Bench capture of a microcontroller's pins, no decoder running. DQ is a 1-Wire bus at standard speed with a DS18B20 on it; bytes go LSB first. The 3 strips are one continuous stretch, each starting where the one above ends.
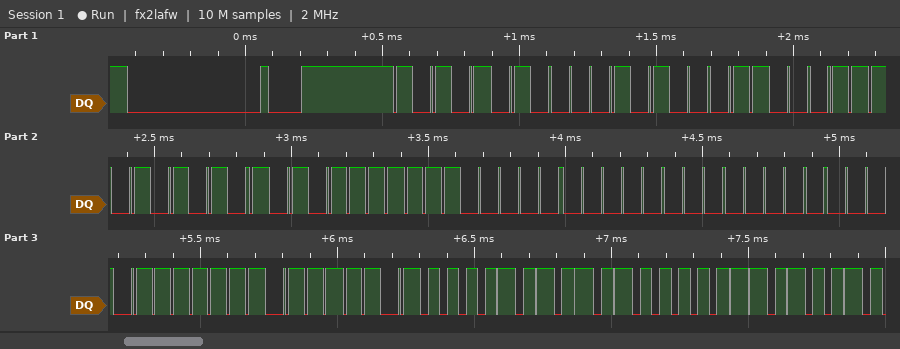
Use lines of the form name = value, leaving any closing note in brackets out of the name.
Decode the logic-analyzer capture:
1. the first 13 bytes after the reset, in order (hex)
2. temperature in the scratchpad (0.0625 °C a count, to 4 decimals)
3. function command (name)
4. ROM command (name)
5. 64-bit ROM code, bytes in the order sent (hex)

the first 13 bytes after the reset, in order = 55 28 C6 55 F5 07 00 00 FE BE 50 05 4B
temperature in the scratchpad = 85.0000 °C
function command = Read Scratchpad
ROM command = Match ROM
64-bit ROM code, bytes in the order sent = 28 C6 55 F5 07 00 00 FE
